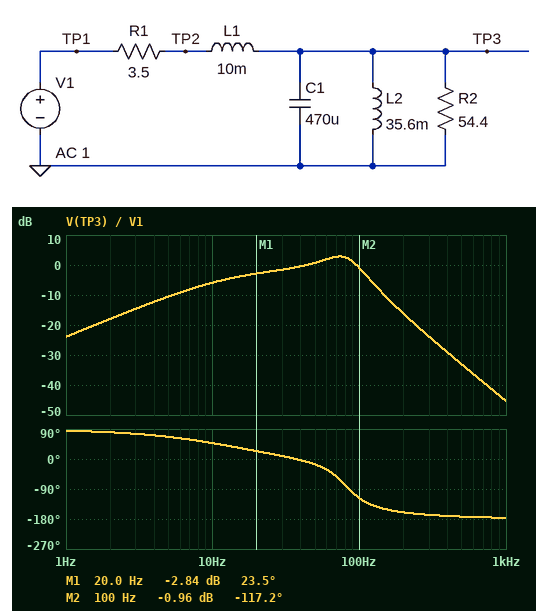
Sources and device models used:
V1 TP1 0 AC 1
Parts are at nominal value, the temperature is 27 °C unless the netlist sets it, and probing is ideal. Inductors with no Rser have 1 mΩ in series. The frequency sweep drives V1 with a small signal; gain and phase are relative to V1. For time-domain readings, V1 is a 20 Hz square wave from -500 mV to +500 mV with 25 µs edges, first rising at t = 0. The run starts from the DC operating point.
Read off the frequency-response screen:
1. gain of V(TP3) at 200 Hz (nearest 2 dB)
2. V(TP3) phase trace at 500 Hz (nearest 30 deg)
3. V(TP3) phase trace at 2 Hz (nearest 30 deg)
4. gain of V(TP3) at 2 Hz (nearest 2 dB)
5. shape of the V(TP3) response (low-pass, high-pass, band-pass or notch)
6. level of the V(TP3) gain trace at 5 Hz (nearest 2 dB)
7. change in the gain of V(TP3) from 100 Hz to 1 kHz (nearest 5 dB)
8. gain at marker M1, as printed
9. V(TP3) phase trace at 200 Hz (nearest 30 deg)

-16 dB
-180 deg
90 deg
-18 dB
band-pass
-10 dB
-45 dB
-2.84 dB
-150 deg
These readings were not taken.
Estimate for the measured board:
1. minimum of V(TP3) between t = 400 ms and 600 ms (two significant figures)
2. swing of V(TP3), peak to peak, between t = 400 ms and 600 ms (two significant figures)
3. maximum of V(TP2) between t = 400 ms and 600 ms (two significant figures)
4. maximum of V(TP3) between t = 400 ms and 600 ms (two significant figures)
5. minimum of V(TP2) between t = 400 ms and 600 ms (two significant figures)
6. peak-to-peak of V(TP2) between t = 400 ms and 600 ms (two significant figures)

-800 mV
1.6 V
860 mV
800 mV
-860 mV
1.7 V
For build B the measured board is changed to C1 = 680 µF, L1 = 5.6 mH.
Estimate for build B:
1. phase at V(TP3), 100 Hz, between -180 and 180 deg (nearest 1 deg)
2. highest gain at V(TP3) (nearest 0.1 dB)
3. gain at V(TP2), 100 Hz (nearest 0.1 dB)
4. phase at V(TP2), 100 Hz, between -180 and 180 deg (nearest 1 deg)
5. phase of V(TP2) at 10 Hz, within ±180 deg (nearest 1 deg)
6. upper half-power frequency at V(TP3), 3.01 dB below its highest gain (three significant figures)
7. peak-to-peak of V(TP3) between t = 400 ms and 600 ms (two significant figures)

-101 deg
0.4 dB
-12.2 dB
68 deg
50 deg
96.4 Hz
1.5 V
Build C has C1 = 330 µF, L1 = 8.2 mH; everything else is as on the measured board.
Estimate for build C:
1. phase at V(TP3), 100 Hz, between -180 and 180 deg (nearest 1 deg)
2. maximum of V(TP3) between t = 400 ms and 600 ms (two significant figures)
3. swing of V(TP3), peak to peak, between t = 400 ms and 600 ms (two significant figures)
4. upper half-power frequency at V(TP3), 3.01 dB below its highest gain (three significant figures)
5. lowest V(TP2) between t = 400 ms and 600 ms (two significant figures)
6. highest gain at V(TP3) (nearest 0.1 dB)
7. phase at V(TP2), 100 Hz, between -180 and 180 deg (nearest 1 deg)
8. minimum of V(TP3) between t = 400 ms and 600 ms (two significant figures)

-71 deg
870 mV
1.7 V
126 Hz
-870 mV
3.1 dB
-41 deg
-870 mV
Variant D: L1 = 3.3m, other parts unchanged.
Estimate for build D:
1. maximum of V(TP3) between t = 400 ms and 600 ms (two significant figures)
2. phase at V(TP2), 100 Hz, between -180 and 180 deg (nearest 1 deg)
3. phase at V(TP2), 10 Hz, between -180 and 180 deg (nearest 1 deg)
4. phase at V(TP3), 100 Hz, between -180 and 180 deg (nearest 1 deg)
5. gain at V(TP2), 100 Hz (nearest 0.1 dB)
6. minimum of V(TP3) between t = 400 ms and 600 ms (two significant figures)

790 mV
-55 deg
52 deg
-59 deg
-6.9 dB
-790 mV
